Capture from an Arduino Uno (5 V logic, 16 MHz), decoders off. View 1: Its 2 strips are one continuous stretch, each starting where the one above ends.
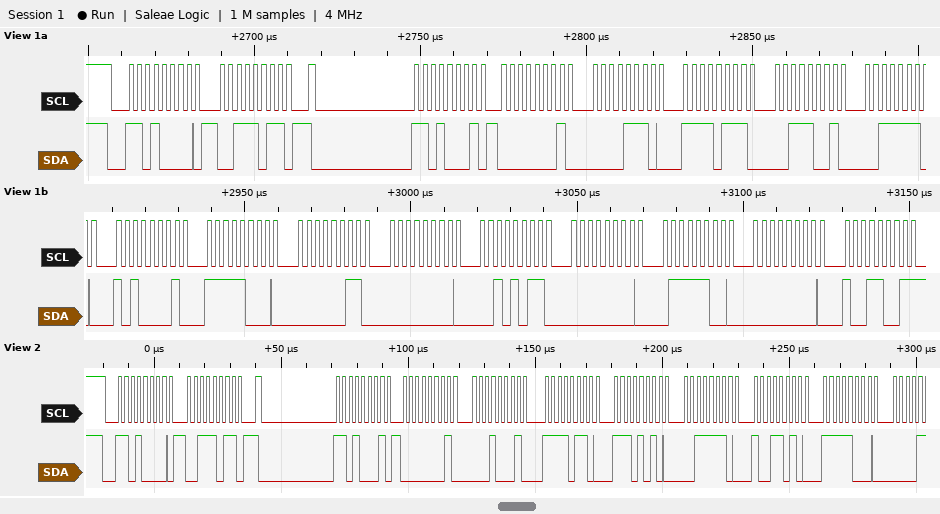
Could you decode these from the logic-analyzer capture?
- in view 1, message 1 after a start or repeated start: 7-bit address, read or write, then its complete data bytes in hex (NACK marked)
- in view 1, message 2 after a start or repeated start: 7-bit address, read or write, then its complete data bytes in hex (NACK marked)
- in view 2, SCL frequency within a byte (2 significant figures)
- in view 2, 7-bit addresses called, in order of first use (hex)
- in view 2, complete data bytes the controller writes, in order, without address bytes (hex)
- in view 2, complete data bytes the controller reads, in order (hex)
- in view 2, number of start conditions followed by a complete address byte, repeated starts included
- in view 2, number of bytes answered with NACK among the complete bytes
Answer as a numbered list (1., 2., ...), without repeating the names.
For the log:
1. 0x68 write: 3B
2. 0x68 read: 01 0E F7 39 3E A1 F8 03 00 2B 00 7C 00 99 NACK
3. 400 kHz
4. 0x68
5. 3B
6. 01 11 F6 EA 3E 9A F8
7. 2
8. 0
